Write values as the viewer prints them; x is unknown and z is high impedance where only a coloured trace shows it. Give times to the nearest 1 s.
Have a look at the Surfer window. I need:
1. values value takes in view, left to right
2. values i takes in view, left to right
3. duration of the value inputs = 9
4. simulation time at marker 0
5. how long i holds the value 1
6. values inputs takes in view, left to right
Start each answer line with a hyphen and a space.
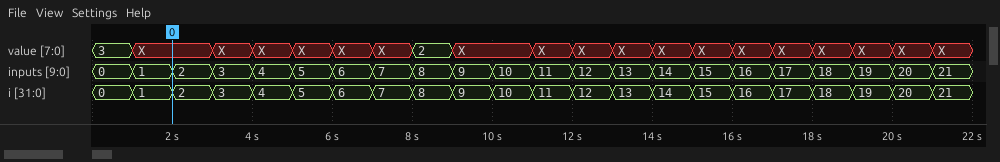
- 3, X, X, X, X, X, X, 2, X, X, X, X, X, X, X, X, X, X, X, X
- 0, 1, 2, 3, 4, 5, 6, 7, 8, 9, 10, 11, 12, 13, 14, 15, 16, 17, 18, 19, 20, 21
- 1 s
- 2 s
- 1 s
- 0, 1, 2, 3, 4, 5, 6, 7, 8, 9, 10, 11, 12, 13, 14, 15, 16, 17, 18, 19, 20, 21
